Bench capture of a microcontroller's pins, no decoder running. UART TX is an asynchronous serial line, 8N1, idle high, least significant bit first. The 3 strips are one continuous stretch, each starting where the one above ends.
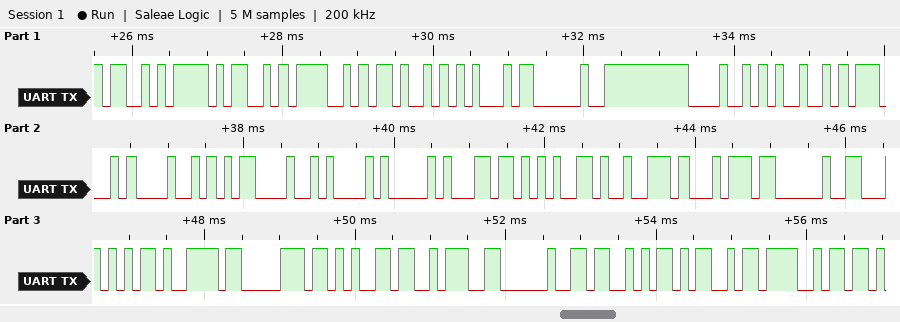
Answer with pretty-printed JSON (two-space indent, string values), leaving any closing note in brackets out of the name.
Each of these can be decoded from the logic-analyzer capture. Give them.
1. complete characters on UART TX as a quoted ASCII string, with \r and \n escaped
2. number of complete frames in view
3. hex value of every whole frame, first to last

{
  "complete characters on UART TX as a quoted ASCII string, with \\r and \\n escaped": "\"SMOKE HIGH\\r\\nAlert Type: SMO\"",
  "number of complete frames in view": "27",
  "hex value of every whole frame, first to last": "53 4D 4F 4B 45 20 48 49 47 48 0D 0A 41 6C 65 72 74 20 54 79 70 65 3A 20 53 4D 4F"
}
